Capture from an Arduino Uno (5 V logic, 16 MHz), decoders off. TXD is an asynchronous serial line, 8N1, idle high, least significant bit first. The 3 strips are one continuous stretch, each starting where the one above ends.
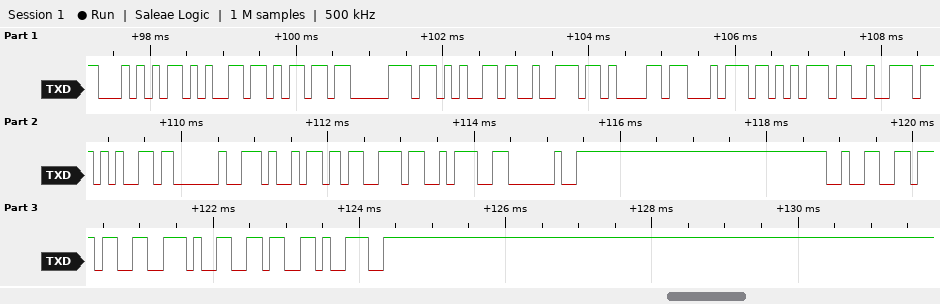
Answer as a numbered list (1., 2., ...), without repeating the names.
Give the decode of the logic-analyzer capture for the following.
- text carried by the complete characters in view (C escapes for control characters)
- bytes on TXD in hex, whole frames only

1. "Temperature is: 27.69"
2. 54 65 6D 70 65 72 61 74 75 72 65 20 69 73 3A 20 32 37 2E 36 39
